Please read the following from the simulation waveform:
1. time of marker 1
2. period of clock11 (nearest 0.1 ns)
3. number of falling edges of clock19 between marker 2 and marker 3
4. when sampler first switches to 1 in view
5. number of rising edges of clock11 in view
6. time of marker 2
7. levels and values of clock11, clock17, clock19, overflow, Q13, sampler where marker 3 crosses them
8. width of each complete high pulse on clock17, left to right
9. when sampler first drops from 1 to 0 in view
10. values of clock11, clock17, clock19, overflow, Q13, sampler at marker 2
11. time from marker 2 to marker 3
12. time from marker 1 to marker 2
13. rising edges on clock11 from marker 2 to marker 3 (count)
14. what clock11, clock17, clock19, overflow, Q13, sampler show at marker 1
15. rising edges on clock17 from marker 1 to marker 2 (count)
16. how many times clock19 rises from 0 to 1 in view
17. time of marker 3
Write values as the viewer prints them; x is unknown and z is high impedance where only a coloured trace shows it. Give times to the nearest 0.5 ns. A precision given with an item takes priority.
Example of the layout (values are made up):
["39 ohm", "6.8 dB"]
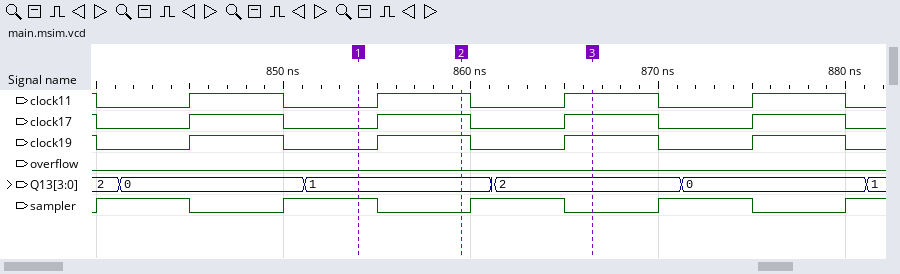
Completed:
["854 ns", "10 ns", "1", "840 ns", "4", "859.5 ns", "clock11=1, clock17=1, clock19=1, overflow=0, Q13=2, sampler=0", "5 ns, 5 ns, 5 ns, 5 ns", "845 ns", "clock11=1, clock17=1, clock19=1, overflow=0, Q13=1, sampler=0", "7 ns", "5.5 ns", "1", "clock11=0, clock17=0, clock19=0, overflow=0, Q13=1, sampler=1", "1", "4", "866.5 ns"]
